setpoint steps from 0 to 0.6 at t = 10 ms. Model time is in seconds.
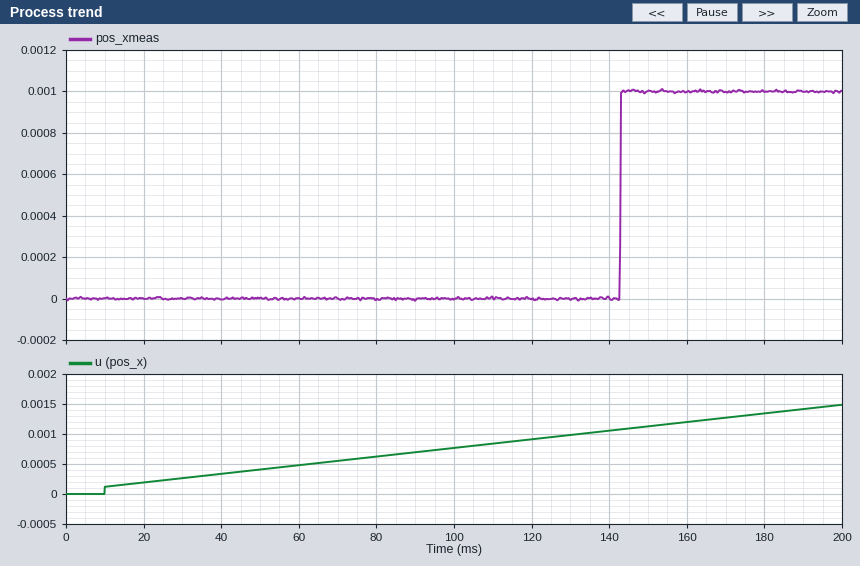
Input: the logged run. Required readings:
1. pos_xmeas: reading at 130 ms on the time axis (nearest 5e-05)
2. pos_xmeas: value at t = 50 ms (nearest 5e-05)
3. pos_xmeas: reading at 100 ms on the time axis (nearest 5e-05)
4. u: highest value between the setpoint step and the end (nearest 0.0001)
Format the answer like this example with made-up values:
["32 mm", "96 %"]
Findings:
["0.00000", "0.00000", "0.00000", "0.0015"]
